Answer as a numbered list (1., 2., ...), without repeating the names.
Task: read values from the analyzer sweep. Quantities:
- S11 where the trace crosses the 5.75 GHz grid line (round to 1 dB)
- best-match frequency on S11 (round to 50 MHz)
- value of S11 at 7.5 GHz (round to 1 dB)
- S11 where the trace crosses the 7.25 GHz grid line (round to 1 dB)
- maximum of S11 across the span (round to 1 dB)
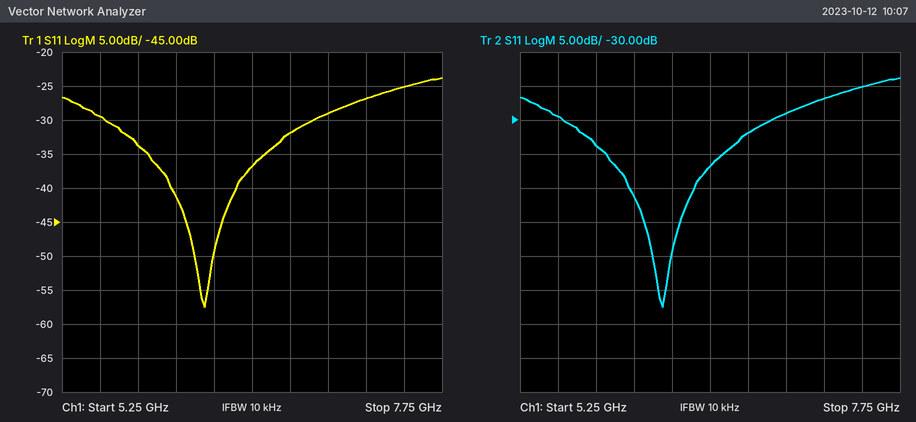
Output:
1. -34 dB
2. 6.20 GHz
3. -25 dB
4. -27 dB
5. -24 dB
